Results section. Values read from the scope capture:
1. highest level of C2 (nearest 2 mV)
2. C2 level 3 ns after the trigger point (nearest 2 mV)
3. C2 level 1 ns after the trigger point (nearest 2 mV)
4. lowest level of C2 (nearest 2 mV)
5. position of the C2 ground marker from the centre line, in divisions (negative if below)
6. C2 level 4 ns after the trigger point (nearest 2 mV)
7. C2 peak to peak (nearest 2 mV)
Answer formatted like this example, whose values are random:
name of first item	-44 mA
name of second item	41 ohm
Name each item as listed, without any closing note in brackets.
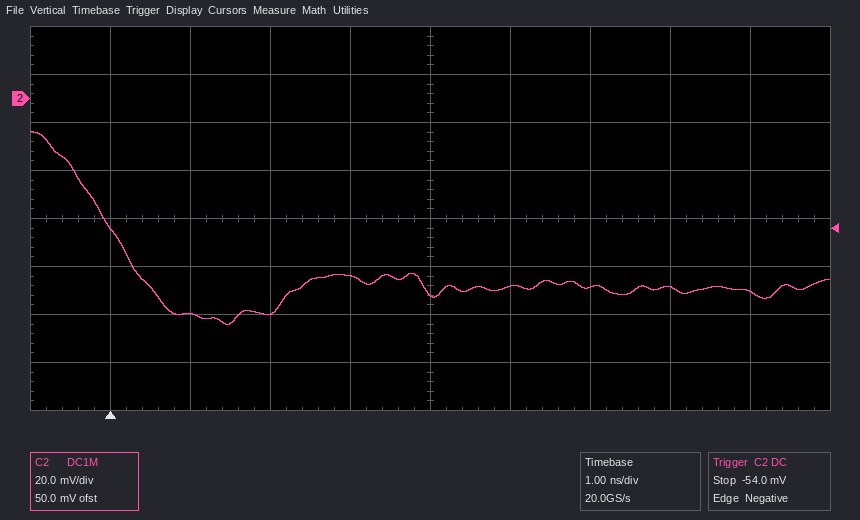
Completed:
highest level of C2	-14 mV
C2 level 3 ns after the trigger point	-74 mV
C2 level 1 ns after the trigger point	-90 mV
lowest level of C2	-94 mV
position of the C2 ground marker from the centre line, in divisions	+2.5 div
C2 level 4 ns after the trigger point	-82 mV
C2 peak to peak	80 mV
